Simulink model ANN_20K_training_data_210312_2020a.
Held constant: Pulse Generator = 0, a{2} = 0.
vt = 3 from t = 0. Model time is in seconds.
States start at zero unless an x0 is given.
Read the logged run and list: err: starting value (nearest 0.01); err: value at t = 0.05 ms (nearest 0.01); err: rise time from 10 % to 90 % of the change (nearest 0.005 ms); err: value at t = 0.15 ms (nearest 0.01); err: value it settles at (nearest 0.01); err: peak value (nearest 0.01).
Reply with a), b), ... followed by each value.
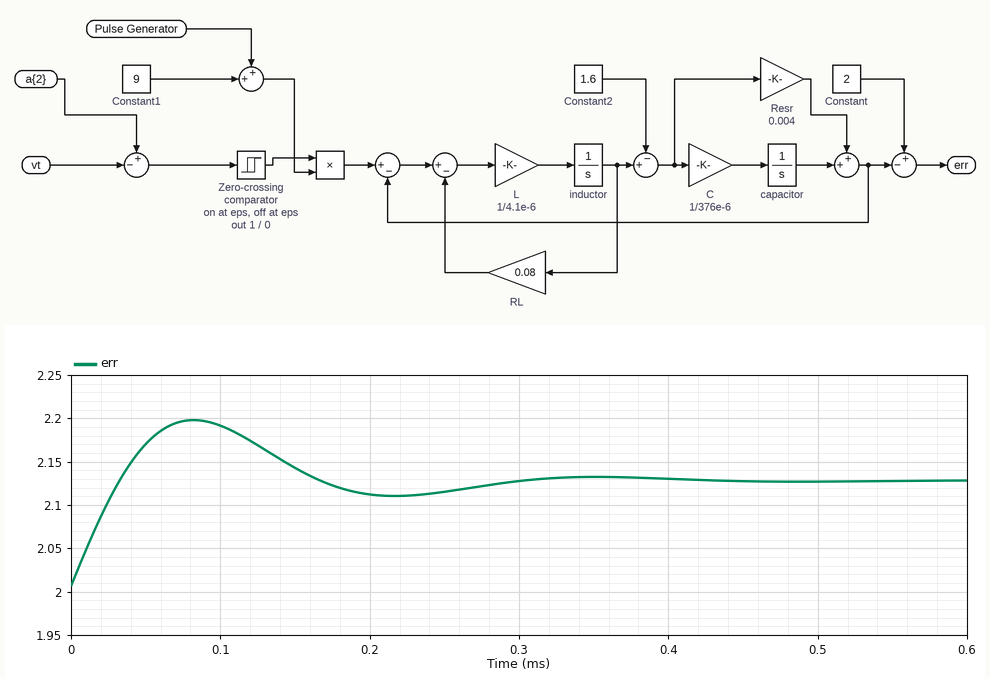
a) 2.01
b) 2.17
c) 0.025 ms
d) 2.14
e) 2.13
f) 2.20
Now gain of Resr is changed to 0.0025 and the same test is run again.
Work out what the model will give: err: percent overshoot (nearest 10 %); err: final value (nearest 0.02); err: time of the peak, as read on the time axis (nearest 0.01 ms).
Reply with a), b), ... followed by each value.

a) 60 %
b) 2.12
c) 0.08 ms
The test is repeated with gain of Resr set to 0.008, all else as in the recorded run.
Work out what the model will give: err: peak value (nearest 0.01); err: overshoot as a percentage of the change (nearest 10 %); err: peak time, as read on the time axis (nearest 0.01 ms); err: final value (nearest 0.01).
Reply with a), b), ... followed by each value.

a) 2.19
b) 60 %
c) 0.08 ms
d) 2.13
